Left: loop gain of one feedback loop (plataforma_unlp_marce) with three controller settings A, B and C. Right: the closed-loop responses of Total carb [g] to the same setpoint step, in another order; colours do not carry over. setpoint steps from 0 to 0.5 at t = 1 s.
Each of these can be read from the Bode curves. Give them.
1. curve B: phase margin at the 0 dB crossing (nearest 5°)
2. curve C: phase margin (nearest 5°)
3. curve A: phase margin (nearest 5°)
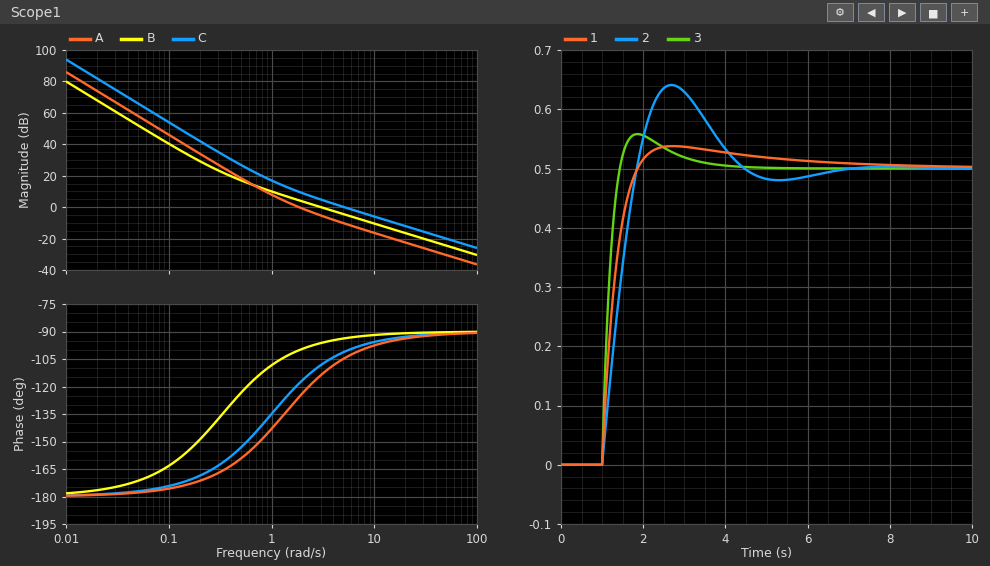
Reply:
85°
80°
55°
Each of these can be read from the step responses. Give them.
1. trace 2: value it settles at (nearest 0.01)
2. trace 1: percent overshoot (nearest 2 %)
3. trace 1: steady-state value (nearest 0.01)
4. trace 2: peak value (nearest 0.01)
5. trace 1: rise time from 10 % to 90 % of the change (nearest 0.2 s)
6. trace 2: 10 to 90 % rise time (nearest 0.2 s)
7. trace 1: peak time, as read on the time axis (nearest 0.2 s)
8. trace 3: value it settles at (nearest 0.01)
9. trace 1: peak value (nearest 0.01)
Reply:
0.50
8 %
0.50
0.64
0.6 s
0.6 s
2.8 s
0.50
0.54
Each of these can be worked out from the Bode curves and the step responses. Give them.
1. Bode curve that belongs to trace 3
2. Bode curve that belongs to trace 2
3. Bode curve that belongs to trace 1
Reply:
C
A
B
